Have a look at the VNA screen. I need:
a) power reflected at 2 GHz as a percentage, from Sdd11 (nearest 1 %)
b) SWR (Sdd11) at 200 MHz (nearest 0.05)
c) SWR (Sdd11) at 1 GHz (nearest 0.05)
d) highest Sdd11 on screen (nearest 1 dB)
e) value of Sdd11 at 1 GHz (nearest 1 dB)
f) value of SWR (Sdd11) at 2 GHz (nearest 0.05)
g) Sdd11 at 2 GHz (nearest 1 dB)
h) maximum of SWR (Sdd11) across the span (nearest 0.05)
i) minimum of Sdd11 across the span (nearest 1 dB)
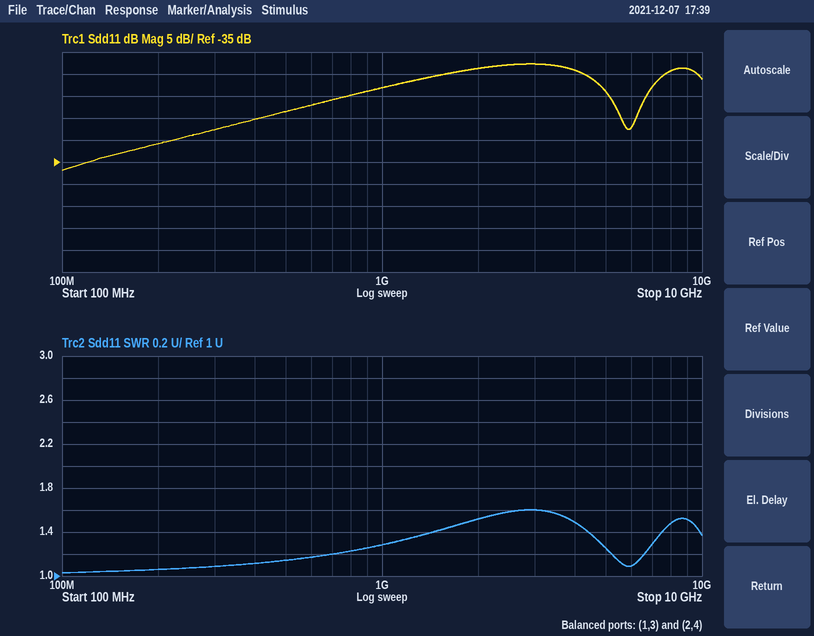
4 %
1.05
1.30
-13 dB
-18 dB
1.50
-14 dB
1.60
-37 dB
